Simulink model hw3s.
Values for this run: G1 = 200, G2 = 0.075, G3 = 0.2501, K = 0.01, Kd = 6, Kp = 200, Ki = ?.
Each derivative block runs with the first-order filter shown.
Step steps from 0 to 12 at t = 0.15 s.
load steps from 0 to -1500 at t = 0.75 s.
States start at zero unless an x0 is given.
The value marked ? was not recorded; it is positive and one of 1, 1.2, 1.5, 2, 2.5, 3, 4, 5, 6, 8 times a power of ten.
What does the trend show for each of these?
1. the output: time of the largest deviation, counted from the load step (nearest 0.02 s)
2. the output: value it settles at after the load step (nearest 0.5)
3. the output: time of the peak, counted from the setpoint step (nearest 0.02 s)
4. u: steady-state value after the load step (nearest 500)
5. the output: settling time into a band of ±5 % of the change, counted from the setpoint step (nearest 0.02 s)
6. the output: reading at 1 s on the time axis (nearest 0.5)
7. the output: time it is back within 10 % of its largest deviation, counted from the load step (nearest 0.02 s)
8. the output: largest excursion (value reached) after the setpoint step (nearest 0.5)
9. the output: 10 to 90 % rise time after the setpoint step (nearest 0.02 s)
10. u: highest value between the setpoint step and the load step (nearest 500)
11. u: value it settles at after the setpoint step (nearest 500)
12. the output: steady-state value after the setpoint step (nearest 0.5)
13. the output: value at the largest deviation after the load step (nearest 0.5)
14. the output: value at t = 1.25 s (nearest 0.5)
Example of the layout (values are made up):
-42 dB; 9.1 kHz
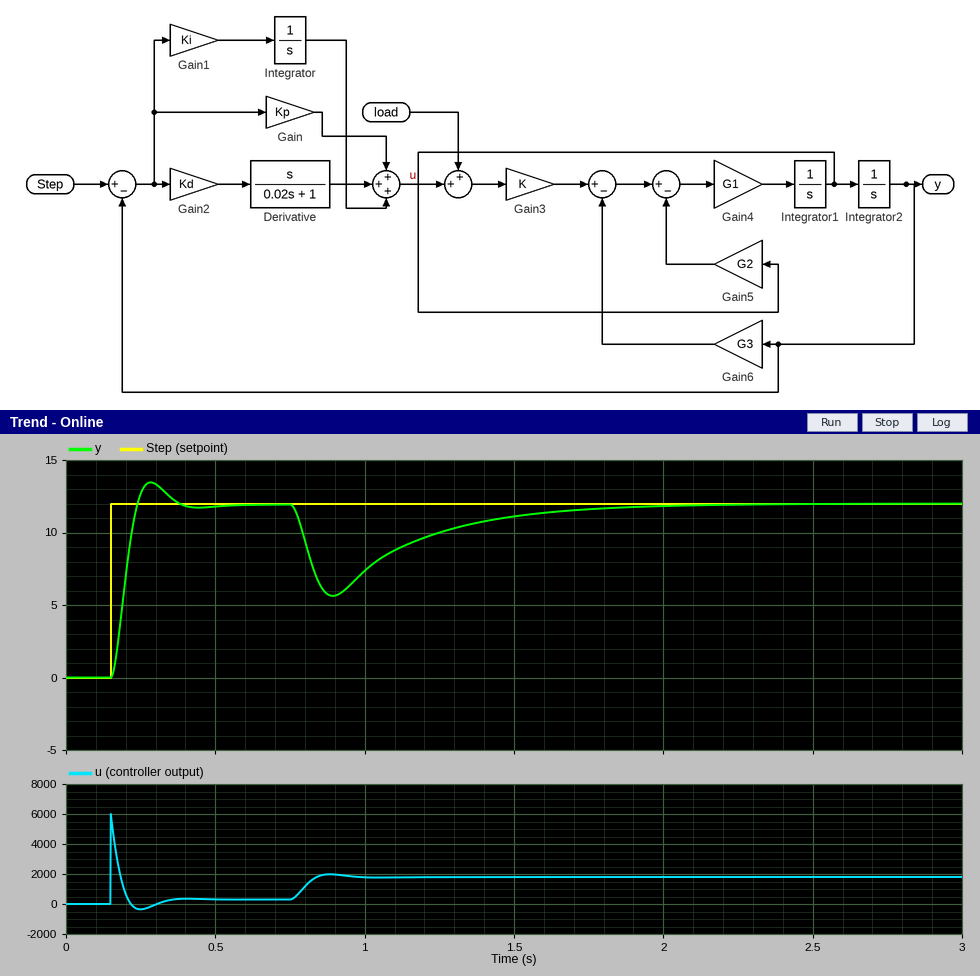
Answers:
0.14 s; 12.0; 0.14 s; 2000; 0.20 s; 7.5; 0.86 s; 13.5; 0.06 s; 6000; 500; 12.0; 5.5; 10.0
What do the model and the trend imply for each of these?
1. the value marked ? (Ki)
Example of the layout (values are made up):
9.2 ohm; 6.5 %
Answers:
600
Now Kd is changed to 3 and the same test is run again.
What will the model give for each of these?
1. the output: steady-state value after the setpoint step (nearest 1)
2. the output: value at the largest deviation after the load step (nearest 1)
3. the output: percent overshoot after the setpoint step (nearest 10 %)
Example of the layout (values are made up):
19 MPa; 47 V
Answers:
12; 5; 20 %
